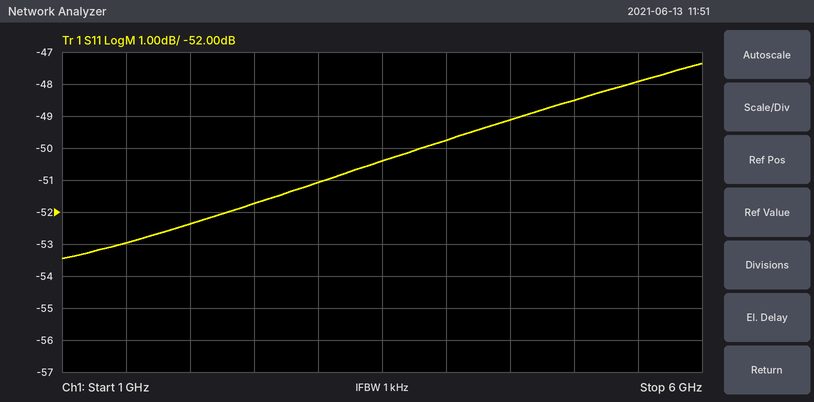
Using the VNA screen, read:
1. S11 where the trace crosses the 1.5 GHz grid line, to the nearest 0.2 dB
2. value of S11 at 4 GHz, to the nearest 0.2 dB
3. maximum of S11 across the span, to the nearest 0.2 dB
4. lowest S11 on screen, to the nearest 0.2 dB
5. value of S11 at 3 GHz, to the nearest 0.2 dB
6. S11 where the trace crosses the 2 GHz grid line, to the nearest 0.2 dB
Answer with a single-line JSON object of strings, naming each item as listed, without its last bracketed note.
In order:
{"S11 where the trace crosses the 1.5 GHz grid line, to the nearest 0.2 dB": "-53.0 dB", "value of S11 at 4 GHz, to the nearest 0.2 dB": "-49.8 dB", "maximum of S11 across the span, to the nearest 0.2 dB": "-47.4 dB", "lowest S11 on screen, to the nearest 0.2 dB": "-53.4 dB", "value of S11 at 3 GHz, to the nearest 0.2 dB": "-51.0 dB", "S11 where the trace crosses the 2 GHz grid line, to the nearest 0.2 dB": "-52.4 dB"}
